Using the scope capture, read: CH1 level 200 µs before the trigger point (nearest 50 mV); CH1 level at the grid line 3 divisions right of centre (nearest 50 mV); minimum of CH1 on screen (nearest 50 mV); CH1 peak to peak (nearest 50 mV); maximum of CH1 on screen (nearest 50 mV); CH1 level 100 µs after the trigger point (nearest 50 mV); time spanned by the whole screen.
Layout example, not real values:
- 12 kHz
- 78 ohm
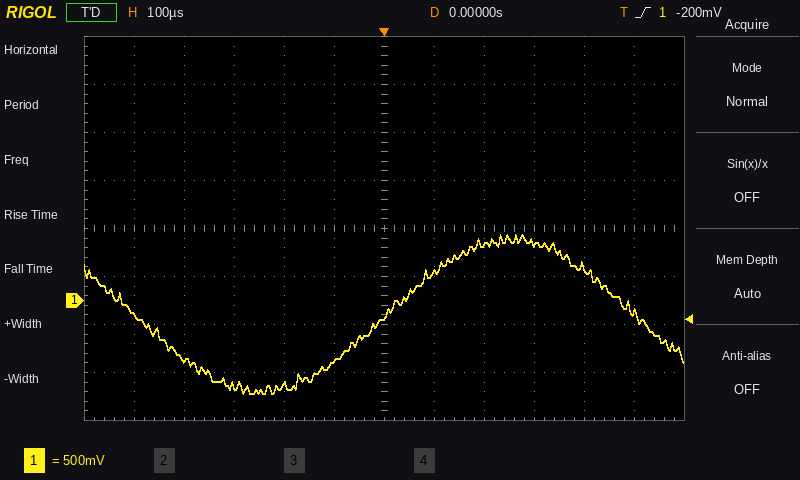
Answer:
- -900 mV
- 600 mV
- -950 mV
- 1.65 V
- 700 mV
- 300 mV
- 1.2 ms
